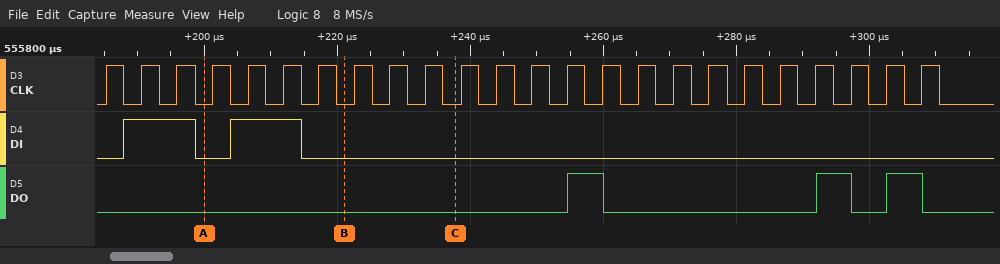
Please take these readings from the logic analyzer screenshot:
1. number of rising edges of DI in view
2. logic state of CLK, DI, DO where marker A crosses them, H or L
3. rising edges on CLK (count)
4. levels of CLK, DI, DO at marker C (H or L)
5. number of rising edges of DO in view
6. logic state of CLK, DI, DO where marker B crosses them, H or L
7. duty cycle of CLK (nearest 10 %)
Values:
2
CLK=L, DI=L, DO=L
24
CLK=L, DI=L, DO=L
3
CLK=L, DI=L, DO=L
50 %
